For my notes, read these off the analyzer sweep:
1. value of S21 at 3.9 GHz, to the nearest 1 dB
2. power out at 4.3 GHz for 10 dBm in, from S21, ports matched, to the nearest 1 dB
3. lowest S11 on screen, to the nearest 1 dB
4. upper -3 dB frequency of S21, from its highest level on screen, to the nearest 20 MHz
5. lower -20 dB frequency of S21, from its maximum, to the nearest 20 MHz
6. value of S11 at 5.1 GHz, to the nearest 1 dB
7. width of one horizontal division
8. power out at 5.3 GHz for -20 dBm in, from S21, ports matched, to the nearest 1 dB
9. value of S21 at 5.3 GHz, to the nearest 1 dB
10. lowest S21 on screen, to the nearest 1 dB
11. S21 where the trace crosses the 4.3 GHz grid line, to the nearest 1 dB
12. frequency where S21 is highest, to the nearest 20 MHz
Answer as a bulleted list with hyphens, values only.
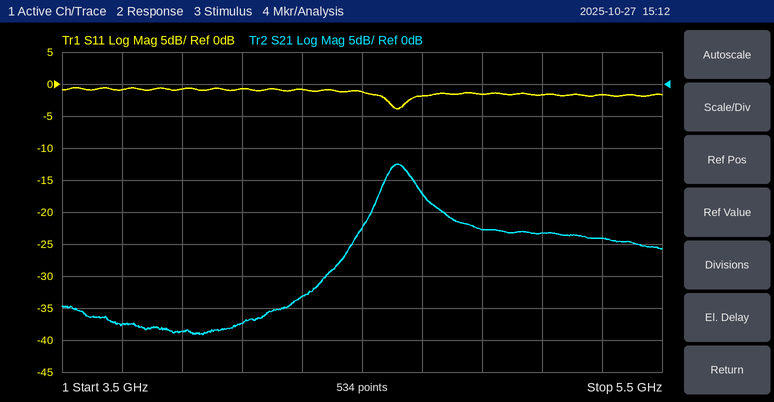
- -39 dB
- -23 dBm
- -4 dB
- 4.68 GHz
- 4.32 GHz
- -2 dB
- 200 MHz
- -44 dBm
- -24 dB
- -39 dB
- -33 dB
- 4.62 GHz
